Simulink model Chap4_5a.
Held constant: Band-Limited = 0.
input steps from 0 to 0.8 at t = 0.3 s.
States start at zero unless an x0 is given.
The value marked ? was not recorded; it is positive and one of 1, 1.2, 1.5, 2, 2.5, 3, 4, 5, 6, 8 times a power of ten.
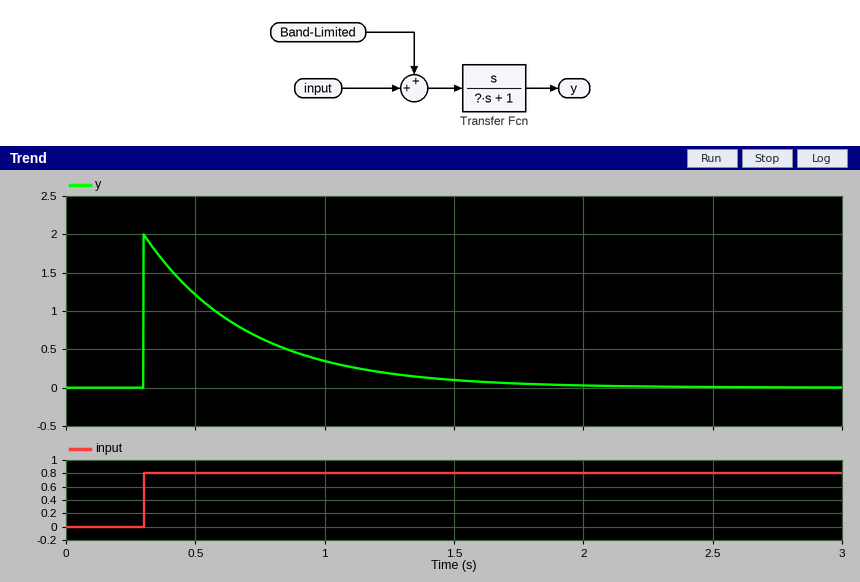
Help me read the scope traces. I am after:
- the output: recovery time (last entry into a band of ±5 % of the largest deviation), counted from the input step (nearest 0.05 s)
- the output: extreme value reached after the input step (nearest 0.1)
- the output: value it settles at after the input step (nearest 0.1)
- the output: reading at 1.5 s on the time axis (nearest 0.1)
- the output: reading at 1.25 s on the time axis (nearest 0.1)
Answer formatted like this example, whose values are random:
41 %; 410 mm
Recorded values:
1.20 s; 2.0; 0.0; 0.1; 0.2
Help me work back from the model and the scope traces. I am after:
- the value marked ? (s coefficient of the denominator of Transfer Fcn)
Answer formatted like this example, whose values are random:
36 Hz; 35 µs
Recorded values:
0.4
